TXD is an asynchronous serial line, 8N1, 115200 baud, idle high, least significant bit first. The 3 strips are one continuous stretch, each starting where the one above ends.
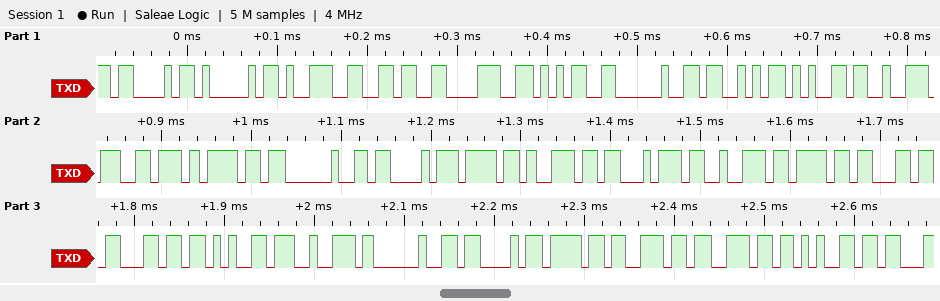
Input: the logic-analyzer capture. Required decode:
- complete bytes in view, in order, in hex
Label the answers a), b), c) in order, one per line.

a) 43 41 39 36 38 35 20 53 65 72 76 6F 20 43 6F 6E 74 72 6F 6C 6C 65 72 20 43 6F 6E 6E 65
